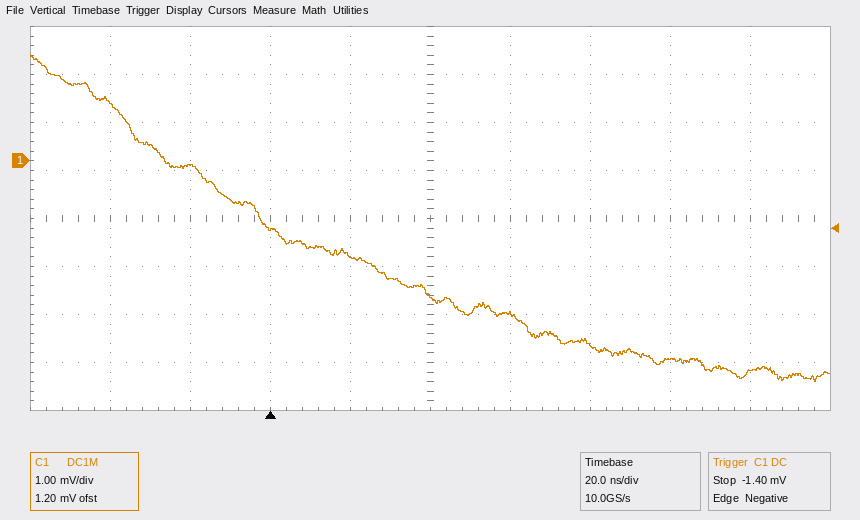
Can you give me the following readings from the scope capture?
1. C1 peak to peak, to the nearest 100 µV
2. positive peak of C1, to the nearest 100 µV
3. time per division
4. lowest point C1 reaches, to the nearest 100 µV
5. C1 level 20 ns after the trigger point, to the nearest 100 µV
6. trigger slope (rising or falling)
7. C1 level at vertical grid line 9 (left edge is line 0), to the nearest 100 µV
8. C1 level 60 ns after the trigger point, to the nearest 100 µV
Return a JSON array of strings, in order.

["6.8 mV", "2.2 mV", "20 ns", "-4.6 mV", "-2.0 mV", "falling", "-4.4 mV", "-3.2 mV"]
